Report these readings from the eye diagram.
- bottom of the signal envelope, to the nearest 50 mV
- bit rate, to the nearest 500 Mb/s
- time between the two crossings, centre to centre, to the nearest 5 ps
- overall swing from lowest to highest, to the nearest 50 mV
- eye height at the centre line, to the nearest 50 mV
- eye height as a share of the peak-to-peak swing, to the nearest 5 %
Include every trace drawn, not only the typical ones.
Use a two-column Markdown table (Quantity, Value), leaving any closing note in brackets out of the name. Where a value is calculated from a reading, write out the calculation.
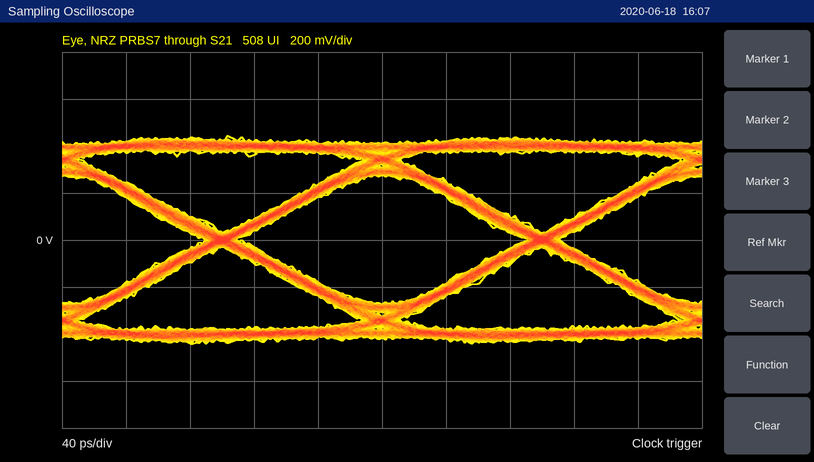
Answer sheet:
| Quantity | Value |
|---|---|
| bottom of the signal envelope, to the nearest 50 mV | -450 mV |
| bit rate, to the nearest 500 Mb/s | 5.0 Gb/s |
| time between the two crossings, centre to centre, to the nearest 5 ps | 200 ps |
| overall swing from lowest to highest, to the nearest 50 mV | 900 mV |
| eye height at the centre line, to the nearest 50 mV | 550 mV |
| eye height as a share of the peak-to-peak swing, to the nearest 5 % | 550 mV / 900 mV ≈ 61.1 %, so 60 % to the nearest 5 % |
